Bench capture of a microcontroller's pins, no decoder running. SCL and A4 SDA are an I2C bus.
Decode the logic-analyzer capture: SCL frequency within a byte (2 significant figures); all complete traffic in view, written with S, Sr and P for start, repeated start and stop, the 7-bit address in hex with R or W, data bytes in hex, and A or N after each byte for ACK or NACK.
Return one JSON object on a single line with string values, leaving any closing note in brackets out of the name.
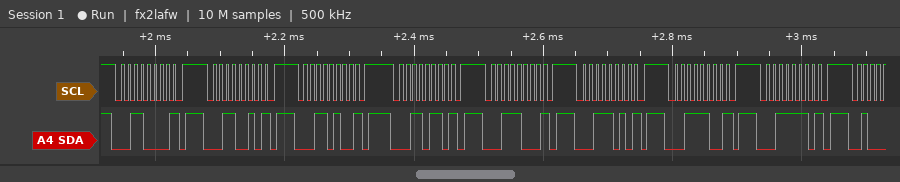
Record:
{"SCL frequency within a byte": "100 kHz", "all complete traffic in view, written with S, Sr and P for start, repeated start and stop, the 7-bit address in hex with R or W, data bytes in hex, and A or N after each byte for ACK or NACK": "S 18W N P S 19W N P S 1AW N P S 1BW N P S 1CW N P S 1DW N P S 1EW N P S 1FW N P"}
